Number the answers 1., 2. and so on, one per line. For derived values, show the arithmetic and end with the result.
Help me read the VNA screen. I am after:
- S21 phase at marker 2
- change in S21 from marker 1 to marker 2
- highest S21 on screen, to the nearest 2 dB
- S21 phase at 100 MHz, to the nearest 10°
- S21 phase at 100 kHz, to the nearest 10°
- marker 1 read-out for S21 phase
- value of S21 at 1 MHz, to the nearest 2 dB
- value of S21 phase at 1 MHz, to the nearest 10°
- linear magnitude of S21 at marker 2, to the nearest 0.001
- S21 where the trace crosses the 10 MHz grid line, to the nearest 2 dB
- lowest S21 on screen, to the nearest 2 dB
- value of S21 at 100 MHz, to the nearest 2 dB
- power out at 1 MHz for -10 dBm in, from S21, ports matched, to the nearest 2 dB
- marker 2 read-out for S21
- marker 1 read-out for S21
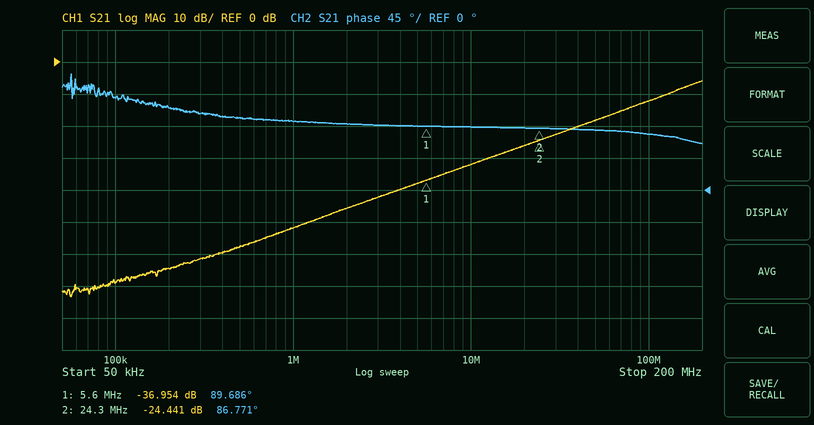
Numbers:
1. 86.771°
2. -24.441 − (-36.954) = 12.513 dB
3. -6 dB
4. 80°
5. 130°
6. 89.686°
7. -52 dB
8. 100°
9. 10^(-24.441/20) ≈ 0.060
10. -32 dB
11. -74 dB
12. -12 dB
13. -10 dBm + (-52 dB) = -62 dBm
14. -24.441 dB
15. -36.954 dB
